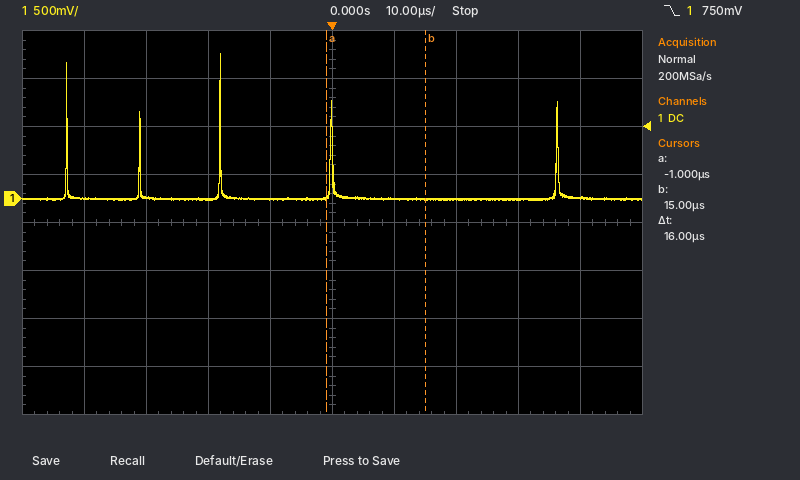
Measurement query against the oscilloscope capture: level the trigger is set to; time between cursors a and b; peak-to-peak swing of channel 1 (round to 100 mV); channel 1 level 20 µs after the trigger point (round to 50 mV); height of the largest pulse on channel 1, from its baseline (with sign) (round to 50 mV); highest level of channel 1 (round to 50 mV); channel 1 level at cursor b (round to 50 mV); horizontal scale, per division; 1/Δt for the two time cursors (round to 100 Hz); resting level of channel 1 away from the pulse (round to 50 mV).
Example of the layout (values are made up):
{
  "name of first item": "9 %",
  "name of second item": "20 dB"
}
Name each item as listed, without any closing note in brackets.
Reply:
{
  "level the trigger is set to": "750 mV",
  "time between cursors a and b": "16 µs",
  "peak-to-peak swing of channel 1": "1.50 V",
  "channel 1 level 20 µs after the trigger point": "0 mV",
  "height of the largest pulse on channel 1, from its baseline (with sign)": "+1.50 V",
  "highest level of channel 1": "1.50 V",
  "channel 1 level at cursor b": "0 mV",
  "horizontal scale, per division": "10 µs",
  "1/Δt for the two time cursors": "62.5 kHz",
  "resting level of channel 1 away from the pulse": "0 mV"
}
